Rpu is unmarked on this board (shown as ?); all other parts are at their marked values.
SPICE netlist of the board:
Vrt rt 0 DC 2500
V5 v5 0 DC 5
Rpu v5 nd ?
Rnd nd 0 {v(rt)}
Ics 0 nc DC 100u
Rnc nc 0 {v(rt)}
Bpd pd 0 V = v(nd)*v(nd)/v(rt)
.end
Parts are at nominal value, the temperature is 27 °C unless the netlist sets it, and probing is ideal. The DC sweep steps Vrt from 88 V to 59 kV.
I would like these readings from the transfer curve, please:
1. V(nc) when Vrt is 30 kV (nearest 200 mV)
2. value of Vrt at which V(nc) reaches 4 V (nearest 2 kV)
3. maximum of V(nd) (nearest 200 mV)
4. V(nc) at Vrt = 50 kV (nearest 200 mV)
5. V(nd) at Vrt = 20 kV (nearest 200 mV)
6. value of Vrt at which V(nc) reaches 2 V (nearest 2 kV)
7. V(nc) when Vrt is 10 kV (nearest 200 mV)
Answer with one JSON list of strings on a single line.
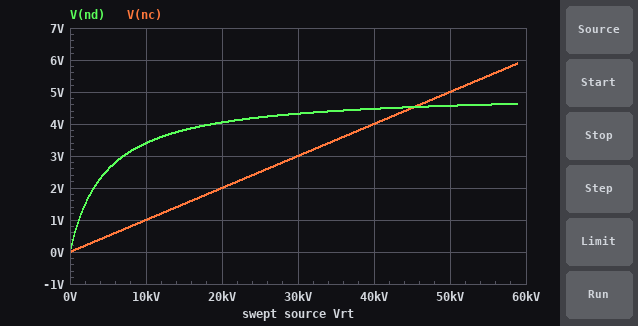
["3.0 V", "40 kV", "4.6 V", "5.0 V", "4.0 V", "20 kV", "1.0 V"]
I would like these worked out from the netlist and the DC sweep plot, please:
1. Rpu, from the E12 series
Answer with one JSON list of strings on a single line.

["4.7 kΩ"]
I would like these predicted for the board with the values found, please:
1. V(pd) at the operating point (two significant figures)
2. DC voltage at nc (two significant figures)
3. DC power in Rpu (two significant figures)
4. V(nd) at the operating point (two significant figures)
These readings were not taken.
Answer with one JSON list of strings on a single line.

["1.2 mV", "250 mV", "2.3 mW", "1.7 V"]
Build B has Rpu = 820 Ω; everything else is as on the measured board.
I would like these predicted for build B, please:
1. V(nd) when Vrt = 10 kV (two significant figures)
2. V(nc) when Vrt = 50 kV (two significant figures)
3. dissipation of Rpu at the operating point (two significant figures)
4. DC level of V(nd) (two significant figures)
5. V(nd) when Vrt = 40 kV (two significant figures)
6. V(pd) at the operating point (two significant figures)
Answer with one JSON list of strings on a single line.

["4.6 V", "5.0 V", "1.9 mW", "3.8 V", "4.9 V", "5.7 mV"]
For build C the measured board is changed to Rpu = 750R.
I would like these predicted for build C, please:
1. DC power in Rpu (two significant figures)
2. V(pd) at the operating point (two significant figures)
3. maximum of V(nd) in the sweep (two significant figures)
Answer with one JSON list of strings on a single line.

["1.8 mW", "5.9 mV", "4.9 V"]
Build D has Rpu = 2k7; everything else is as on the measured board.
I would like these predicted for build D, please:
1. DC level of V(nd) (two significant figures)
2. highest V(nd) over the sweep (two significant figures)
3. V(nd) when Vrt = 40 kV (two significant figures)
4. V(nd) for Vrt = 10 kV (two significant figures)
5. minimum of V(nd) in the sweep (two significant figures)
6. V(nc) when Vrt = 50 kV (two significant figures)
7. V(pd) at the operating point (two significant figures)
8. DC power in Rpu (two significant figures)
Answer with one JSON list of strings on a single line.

["2.4 V", "4.8 V", "4.7 V", "3.9 V", "160 mV", "5.0 V", "2.3 mV", "2.5 mW"]
